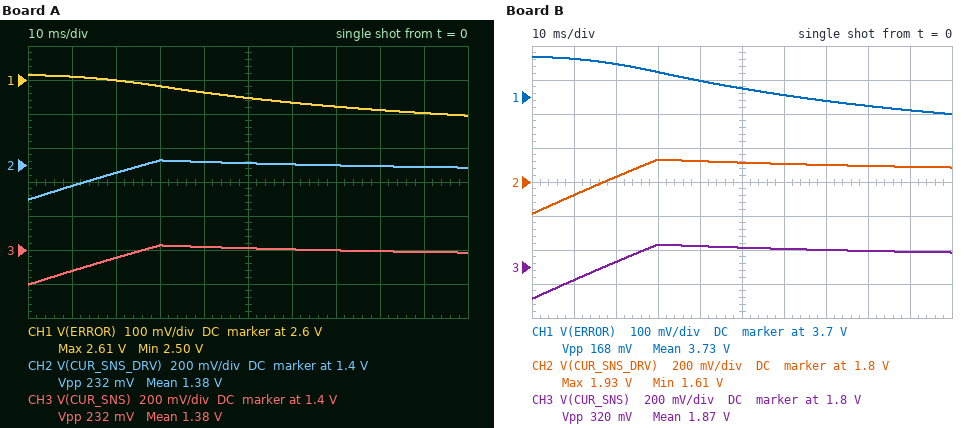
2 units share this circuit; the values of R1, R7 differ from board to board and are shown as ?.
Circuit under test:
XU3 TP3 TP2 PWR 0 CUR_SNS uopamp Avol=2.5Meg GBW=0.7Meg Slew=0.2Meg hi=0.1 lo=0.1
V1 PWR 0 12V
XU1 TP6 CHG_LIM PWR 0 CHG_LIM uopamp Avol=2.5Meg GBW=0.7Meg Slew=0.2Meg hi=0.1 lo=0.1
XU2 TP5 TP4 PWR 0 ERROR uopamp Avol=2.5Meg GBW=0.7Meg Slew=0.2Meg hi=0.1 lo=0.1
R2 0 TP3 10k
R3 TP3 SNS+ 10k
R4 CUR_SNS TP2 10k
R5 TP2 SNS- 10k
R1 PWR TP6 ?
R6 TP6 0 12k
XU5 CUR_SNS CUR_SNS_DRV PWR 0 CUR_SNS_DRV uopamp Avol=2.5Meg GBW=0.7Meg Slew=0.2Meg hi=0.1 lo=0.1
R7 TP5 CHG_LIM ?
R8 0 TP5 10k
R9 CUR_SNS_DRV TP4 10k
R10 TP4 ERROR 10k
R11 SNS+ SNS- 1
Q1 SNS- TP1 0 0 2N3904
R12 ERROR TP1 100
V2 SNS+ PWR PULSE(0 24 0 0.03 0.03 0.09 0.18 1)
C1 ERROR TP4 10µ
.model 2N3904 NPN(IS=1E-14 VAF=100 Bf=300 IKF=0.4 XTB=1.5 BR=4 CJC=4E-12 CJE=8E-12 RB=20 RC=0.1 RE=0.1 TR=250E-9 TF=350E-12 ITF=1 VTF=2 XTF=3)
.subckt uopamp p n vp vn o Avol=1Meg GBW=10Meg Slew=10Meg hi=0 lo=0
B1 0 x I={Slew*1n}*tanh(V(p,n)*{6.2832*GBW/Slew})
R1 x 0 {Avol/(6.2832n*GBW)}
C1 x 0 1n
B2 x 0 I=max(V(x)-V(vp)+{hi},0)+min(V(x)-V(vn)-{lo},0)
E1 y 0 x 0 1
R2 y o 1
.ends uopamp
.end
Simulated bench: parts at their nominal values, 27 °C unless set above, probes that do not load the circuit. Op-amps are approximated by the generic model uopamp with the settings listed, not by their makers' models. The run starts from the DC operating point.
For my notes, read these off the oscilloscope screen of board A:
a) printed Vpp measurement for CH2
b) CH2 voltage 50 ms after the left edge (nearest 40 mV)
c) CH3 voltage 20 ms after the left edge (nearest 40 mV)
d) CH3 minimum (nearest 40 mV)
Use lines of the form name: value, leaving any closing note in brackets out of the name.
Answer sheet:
printed Vpp measurement for CH2: 232 mV
CH2 voltage 50 ms after the left edge: 1.40 V
CH3 voltage 20 ms after the left edge: 1.36 V
CH3 minimum: 1.20 V
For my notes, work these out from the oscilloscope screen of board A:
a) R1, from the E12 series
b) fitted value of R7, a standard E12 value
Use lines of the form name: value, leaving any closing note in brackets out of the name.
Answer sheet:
R1, from the E12 series: 15 kΩ
fitted value of R7, a standard E12 value: 18 kΩ
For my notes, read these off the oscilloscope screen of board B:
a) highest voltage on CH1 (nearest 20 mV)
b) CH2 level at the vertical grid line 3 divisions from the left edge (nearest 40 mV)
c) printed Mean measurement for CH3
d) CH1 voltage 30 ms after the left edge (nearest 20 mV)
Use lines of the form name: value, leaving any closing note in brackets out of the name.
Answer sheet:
highest voltage on CH1: 3.82 V
CH2 level at the vertical grid line 3 divisions from the left edge: 1.92 V
printed Mean measurement for CH3: 1.87 V
CH1 voltage 30 ms after the left edge: 3.78 V
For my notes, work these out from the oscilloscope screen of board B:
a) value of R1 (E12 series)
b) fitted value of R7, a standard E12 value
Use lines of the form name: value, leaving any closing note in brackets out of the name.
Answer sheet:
value of R1: 22 kΩ
fitted value of R7, a standard E12 value: 5.6 kΩ
